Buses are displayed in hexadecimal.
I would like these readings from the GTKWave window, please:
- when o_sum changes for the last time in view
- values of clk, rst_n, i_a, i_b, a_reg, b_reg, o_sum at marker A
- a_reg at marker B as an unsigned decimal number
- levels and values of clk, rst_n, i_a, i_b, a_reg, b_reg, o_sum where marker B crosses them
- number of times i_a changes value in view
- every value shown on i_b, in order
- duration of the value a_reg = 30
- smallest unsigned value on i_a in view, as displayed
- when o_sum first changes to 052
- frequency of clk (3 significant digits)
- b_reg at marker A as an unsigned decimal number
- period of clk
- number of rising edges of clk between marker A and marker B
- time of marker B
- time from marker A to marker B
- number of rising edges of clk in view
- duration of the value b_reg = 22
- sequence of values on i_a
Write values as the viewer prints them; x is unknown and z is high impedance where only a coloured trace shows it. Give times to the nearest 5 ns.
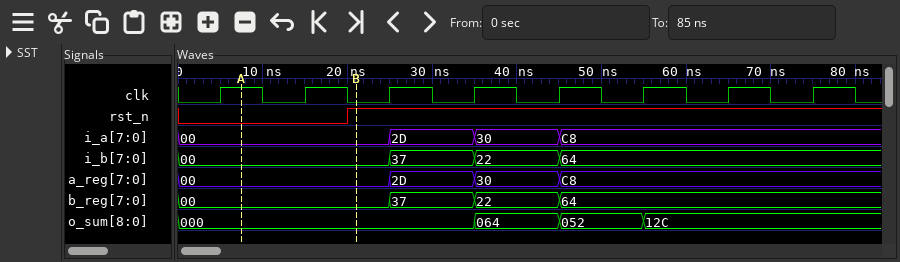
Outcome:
55 ns
clk=1, rst_n=0, i_a=00, i_b=00, a_reg=00, b_reg=00, o_sum=000
0
clk=0, rst_n=1, i_a=00, i_b=00, a_reg=00, b_reg=00, o_sum=000
3
00, 37, 22, 64
10 ns
00
45 ns
100 MHz
0
10 ns
1
20 ns
15 ns
8
10 ns
00, 2D, 30, C8
